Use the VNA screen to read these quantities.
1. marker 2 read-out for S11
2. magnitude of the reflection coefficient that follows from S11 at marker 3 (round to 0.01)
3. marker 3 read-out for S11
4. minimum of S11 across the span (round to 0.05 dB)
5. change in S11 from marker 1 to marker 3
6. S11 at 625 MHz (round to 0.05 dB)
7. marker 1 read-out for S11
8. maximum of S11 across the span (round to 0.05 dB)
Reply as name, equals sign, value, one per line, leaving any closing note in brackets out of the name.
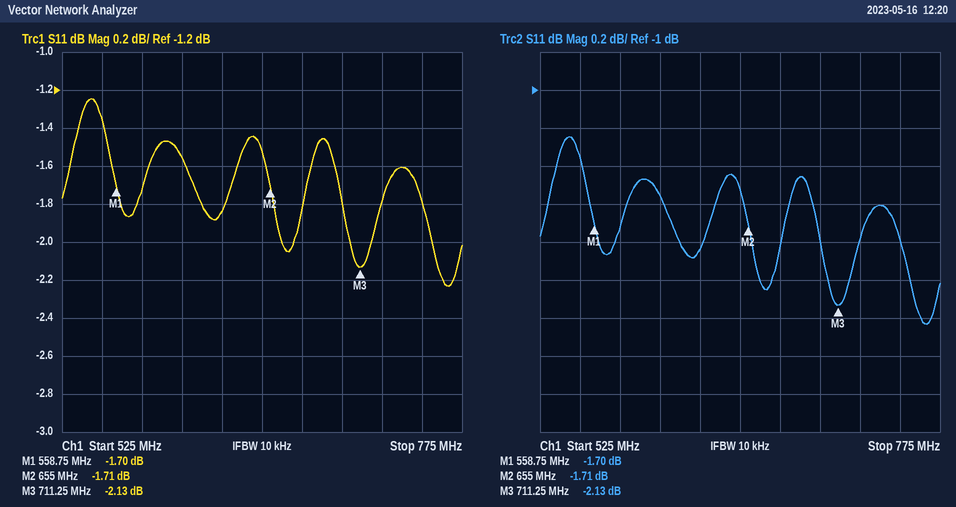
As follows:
marker 2 read-out for S11 = -1.71 dB
magnitude of the reflection coefficient that follows from S11 at marker 3 = 0.78
marker 3 read-out for S11 = -2.13 dB
minimum of S11 across the span = -2.25 dB
change in S11 from marker 1 to marker 3 = -0.43 dB
S11 at 625 MHz = -1.85 dB
marker 1 read-out for S11 = -1.70 dB
maximum of S11 across the span = -1.25 dB
